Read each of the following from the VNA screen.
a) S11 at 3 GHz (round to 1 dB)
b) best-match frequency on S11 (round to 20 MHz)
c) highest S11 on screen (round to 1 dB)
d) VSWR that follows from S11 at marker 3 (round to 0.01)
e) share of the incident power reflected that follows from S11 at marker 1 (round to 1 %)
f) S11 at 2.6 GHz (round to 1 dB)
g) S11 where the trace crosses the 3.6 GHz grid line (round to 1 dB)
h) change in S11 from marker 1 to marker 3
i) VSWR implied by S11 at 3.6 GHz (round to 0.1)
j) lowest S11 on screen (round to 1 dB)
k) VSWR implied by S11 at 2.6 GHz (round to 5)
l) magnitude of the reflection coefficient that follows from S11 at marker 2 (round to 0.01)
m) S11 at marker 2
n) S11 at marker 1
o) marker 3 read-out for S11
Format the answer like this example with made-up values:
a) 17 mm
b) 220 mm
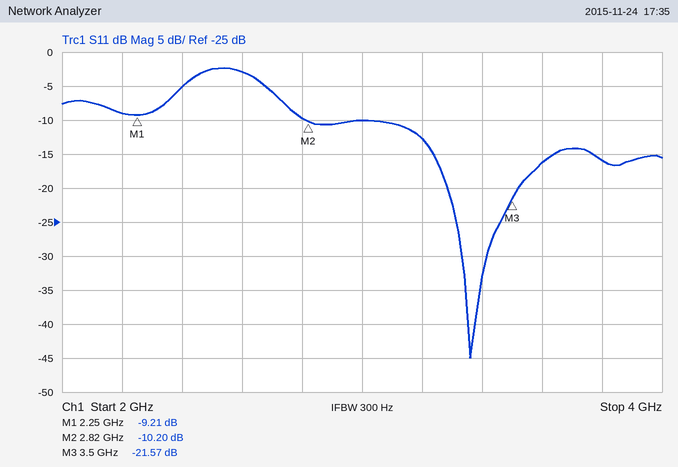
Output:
a) -10 dB
b) 3.36 GHz
c) -2 dB
d) 1.18
e) 12 %
f) -3 dB
g) -16 dB
h) -12.36 dB
i) 1.4
j) -45 dB
k) 5
l) 0.31
m) -10.20 dB
n) -9.21 dB
o) -21.57 dB
